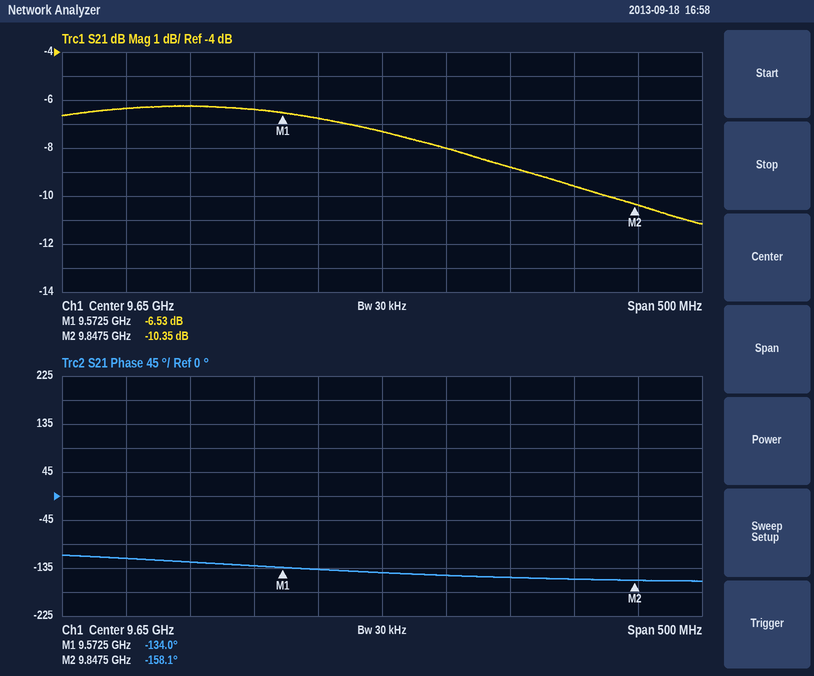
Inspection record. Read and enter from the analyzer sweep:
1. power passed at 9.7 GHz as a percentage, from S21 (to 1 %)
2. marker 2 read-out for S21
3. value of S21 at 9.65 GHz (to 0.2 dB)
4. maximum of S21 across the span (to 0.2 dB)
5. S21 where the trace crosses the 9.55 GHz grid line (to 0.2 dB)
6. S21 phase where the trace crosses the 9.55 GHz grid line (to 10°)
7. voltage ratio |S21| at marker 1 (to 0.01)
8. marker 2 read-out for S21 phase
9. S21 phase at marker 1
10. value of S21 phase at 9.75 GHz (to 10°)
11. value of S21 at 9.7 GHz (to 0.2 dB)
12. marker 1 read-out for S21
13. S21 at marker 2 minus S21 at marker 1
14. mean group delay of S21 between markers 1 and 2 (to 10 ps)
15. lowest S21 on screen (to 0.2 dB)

16 %
-10.35 dB
-7.4 dB
-6.2 dB
-6.4 dB
-130°
0.47
-158.1°
-134.0°
-150°
-8.0 dB
-6.53 dB
-3.82 dB
240 ps
-11.2 dB
